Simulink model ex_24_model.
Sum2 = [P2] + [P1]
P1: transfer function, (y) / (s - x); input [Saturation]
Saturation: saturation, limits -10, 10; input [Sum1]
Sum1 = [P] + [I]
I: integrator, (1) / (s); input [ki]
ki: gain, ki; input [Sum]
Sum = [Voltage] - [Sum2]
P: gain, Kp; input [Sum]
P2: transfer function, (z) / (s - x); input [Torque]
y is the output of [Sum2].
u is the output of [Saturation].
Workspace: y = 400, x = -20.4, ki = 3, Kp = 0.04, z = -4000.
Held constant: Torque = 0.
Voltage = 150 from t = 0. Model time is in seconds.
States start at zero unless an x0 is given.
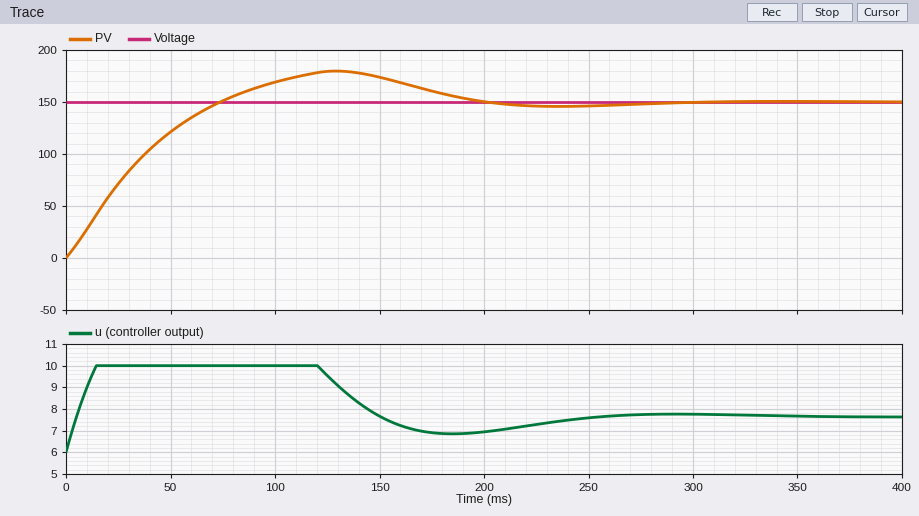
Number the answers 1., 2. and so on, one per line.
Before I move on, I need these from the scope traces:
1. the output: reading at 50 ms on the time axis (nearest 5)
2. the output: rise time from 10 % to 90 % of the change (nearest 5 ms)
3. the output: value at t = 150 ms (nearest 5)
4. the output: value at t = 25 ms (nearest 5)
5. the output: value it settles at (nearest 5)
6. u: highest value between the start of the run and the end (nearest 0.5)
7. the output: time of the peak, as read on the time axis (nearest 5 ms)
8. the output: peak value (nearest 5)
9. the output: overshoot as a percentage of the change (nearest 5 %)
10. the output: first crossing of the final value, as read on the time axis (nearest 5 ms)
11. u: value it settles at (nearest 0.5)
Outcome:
1. 120
2. 55 ms
3. 175
4. 70
5. 150
6. 10.0
7. 130 ms
8. 180
9. 20 %
10. 75 ms
11. 7.5
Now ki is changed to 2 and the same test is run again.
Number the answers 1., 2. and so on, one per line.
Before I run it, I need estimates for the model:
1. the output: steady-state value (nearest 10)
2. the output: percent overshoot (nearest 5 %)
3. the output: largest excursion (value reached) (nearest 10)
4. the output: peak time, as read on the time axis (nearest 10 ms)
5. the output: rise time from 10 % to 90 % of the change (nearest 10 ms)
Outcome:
1. 150
2. 10 %
3. 160
4. 120 ms
5. 60 ms
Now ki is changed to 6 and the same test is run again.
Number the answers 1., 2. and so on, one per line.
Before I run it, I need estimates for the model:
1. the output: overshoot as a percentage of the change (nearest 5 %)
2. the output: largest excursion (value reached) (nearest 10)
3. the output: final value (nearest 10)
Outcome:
1. 25 %
2. 190
3. 150
